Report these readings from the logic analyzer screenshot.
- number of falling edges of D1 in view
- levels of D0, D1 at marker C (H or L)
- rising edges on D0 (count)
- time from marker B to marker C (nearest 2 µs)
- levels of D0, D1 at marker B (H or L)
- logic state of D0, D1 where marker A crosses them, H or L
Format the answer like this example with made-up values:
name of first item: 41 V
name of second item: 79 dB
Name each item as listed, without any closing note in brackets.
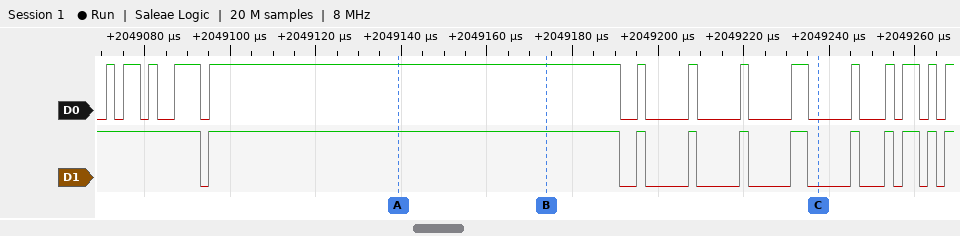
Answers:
number of falling edges of D1 in view: 10
levels of D0, D1 at marker C: D0=L, D1=L
rising edges on D0: 14
time from marker B to marker C: 64 µs
levels of D0, D1 at marker B: D0=H, D1=H
logic state of D0, D1 where marker A crosses them, H or L: D0=H, D1=H
